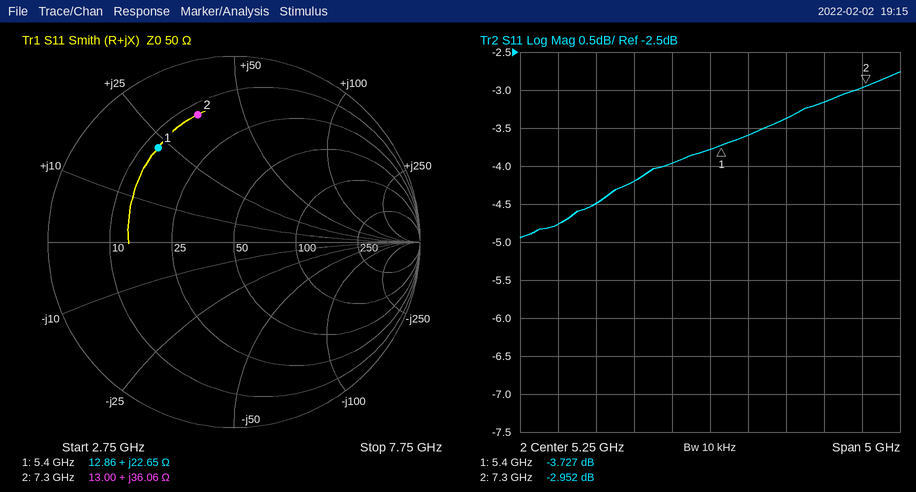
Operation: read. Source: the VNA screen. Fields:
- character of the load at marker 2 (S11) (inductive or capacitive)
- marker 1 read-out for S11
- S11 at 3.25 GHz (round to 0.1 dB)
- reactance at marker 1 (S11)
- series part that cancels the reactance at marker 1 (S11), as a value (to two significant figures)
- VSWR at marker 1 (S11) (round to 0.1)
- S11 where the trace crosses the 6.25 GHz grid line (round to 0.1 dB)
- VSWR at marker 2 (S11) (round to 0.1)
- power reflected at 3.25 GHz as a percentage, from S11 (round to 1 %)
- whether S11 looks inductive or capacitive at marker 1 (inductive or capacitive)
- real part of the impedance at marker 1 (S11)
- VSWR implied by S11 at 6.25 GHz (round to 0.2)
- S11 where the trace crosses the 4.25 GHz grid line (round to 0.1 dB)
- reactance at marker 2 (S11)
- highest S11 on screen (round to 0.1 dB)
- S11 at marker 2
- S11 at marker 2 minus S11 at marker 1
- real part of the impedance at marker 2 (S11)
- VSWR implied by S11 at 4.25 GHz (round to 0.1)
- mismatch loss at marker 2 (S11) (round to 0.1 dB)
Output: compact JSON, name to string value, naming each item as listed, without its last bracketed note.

{"character of the load at marker 2 (S11)": "inductive", "marker 1 read-out for S11": "-3.727 dB", "S11 at 3.25 GHz": "-4.8 dB", "reactance at marker 1": "+22.65 Ω", "series part that cancels the reactance at marker 1 (S11), as a value": "1.3 pF", "VSWR at marker 1 (S11)": "4.7", "S11 where the trace crosses the 6.25 GHz grid line": "-3.4 dB", "VSWR at marker 2 (S11)": "5.9", "power reflected at 3.25 GHz as a percentage, from S11": "33 %", "whether S11 looks inductive or capacitive at marker 1": "inductive", "real part of the impedance at marker 1": "12.86 Ω", "VSWR implied by S11 at 6.25 GHz": "5.2", "S11 where the trace crosses the 4.25 GHz grid line": "-4.2 dB", "reactance at marker 2": "+36.06 Ω", "highest S11 on screen": "-2.8 dB", "S11 at marker 2": "-2.952 dB", "S11 at marker 2 minus S11 at marker 1": "0.775 dB", "real part of the impedance at marker 2": "13.00 Ω", "VSWR implied by S11 at 4.25 GHz": "4.2", "mismatch loss at marker 2 (S11)": "3.1 dB"}
